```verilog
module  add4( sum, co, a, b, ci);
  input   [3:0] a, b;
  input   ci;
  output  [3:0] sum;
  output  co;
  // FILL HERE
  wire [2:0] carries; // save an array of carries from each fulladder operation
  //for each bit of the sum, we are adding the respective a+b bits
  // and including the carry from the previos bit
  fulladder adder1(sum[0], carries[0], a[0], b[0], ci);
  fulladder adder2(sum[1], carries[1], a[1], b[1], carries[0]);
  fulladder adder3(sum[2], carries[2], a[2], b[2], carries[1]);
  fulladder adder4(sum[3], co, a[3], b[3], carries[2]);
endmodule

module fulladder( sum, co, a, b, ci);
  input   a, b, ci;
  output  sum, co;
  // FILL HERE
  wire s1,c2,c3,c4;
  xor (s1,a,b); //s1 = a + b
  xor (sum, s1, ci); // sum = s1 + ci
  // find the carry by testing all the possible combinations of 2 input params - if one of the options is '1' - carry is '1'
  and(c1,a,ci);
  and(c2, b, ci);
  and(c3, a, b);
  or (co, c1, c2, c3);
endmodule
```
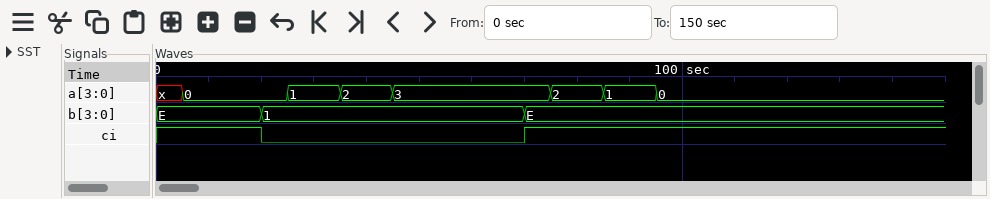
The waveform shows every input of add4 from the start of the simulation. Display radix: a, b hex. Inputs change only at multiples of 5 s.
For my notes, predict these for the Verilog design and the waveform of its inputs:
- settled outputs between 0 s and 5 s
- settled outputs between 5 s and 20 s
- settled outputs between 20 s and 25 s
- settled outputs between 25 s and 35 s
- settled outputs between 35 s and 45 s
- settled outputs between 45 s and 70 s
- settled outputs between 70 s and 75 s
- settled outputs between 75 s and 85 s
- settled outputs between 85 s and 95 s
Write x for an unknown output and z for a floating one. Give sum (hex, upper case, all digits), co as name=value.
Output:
sum=x, co=x
sum=F, co=0
sum=1, co=0
sum=2, co=0
sum=3, co=0
sum=4, co=0
sum=2, co=1
sum=1, co=1
sum=0, co=1
